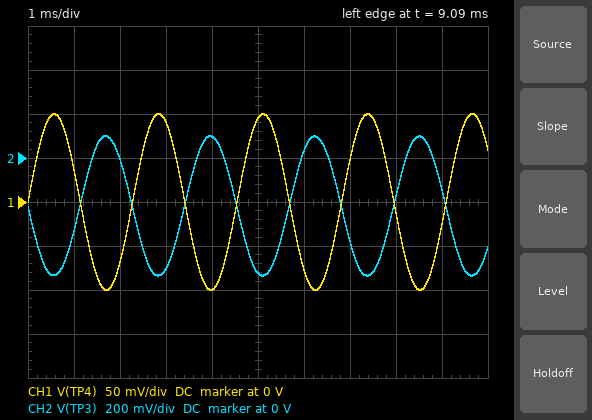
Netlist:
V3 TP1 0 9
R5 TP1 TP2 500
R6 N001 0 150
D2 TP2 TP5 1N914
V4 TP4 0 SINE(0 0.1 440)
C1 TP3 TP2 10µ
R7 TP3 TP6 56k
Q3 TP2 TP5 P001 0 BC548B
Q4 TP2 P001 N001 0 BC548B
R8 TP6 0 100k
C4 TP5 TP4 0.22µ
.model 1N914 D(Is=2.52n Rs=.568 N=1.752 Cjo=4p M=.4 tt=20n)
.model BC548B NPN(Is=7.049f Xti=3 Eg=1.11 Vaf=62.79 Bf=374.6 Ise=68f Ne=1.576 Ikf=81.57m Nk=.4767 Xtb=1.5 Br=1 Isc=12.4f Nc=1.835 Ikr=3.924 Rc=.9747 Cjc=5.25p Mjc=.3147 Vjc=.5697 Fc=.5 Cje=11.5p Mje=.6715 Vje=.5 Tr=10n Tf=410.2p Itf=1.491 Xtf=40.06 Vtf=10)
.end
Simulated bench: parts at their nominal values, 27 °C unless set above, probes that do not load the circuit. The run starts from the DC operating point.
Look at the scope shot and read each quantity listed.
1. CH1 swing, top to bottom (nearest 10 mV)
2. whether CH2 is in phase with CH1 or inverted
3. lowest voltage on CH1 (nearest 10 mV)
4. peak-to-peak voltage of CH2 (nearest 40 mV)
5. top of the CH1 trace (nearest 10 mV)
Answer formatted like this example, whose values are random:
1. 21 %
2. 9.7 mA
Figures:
1. 200 mV
2. inverted
3. -100 mV
4. 640 mV
5. 100 mV
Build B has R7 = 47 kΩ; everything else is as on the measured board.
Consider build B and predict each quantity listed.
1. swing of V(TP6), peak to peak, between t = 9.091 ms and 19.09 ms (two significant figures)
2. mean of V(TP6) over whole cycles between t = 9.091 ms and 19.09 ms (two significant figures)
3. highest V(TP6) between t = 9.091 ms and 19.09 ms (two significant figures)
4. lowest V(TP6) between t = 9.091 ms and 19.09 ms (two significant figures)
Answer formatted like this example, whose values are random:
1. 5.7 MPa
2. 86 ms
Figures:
1. 430 mV
2. -150 mV
3. 68 mV
4. -360 mV
